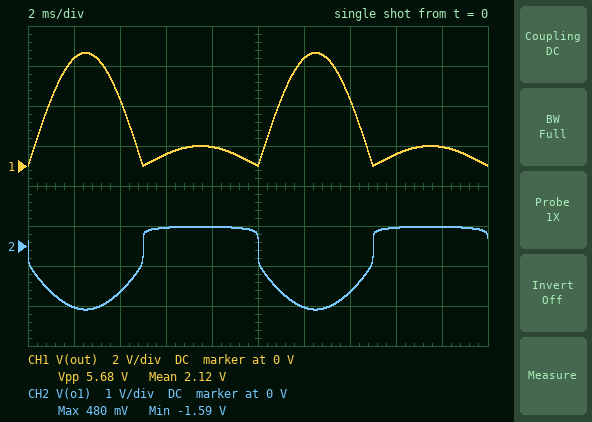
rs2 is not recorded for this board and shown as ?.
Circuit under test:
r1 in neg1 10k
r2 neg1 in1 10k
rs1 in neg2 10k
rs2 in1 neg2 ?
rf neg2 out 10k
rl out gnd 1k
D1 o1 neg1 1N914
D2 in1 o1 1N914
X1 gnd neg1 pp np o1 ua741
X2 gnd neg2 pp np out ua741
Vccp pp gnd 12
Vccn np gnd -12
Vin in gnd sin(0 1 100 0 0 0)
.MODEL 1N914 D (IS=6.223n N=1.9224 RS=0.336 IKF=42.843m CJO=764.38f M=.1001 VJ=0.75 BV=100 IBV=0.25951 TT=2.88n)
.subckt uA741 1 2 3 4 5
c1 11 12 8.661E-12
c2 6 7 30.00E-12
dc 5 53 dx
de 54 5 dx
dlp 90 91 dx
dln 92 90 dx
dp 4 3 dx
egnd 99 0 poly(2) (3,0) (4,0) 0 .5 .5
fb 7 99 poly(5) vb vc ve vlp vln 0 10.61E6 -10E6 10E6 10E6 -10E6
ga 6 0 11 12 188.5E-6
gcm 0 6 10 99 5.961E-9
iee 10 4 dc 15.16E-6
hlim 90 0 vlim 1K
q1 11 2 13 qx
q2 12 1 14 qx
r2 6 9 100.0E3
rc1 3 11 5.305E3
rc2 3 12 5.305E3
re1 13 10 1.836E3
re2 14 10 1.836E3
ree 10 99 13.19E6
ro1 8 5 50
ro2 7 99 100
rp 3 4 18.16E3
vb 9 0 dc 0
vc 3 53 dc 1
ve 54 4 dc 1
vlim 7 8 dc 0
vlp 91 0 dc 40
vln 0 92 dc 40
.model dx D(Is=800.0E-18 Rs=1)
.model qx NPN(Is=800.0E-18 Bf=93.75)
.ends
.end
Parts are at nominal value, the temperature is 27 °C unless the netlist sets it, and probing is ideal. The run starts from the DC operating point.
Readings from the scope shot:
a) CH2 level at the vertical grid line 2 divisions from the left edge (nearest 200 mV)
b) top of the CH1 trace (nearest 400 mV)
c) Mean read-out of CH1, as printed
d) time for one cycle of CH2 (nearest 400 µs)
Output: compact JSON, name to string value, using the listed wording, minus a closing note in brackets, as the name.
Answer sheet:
{"CH2 level at the vertical grid line 2 divisions from the left edge": "-1.2 V", "top of the CH1 trace": "5.6 V", "Mean read-out of CH1, as printed": "2.12 V", "time for one cycle of CH2": "10.0 ms"}
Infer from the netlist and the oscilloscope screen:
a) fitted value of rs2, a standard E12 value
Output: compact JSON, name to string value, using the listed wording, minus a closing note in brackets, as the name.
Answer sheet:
{"fitted value of rs2, a standard E12 value": "1.5 kΩ"}
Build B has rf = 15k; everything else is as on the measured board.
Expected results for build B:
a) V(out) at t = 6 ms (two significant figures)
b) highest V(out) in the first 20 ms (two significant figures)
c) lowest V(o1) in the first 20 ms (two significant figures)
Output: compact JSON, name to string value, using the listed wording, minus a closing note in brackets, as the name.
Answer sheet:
{"V(out) at t = 6 ms": "880 mV", "highest V(out) in the first 20 ms": "8.5 V", "lowest V(o1) in the first 20 ms": "-1.6 V"}
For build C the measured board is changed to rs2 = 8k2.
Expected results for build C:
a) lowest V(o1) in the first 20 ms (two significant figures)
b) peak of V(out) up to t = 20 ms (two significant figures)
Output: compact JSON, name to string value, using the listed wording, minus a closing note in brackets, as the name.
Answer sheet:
{"lowest V(o1) in the first 20 ms": "-1.5 V", "peak of V(out) up to t = 20 ms": "1.0 V"}
